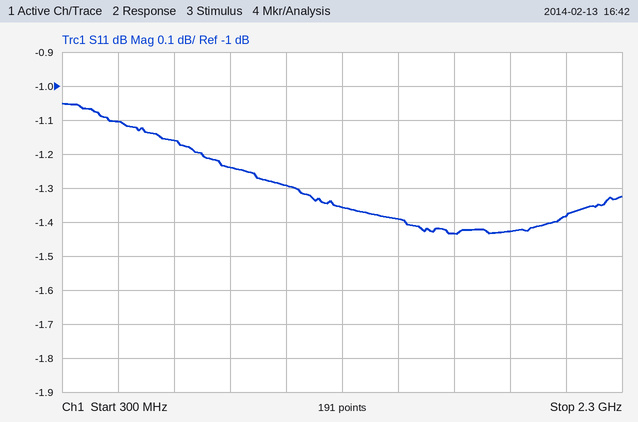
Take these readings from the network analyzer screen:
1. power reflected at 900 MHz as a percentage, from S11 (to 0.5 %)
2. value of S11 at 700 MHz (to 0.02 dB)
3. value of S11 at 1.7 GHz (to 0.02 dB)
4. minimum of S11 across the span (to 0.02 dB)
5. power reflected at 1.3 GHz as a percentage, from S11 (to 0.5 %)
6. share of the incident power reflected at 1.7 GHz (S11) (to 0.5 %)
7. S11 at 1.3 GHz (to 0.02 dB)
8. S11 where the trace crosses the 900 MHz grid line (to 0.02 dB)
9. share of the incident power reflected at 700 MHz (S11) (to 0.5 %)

75.0 %
-1.16 dB
-1.44 dB
-1.44 dB
73.0 %
72.0 %
-1.36 dB
-1.24 dB
76.5 %
